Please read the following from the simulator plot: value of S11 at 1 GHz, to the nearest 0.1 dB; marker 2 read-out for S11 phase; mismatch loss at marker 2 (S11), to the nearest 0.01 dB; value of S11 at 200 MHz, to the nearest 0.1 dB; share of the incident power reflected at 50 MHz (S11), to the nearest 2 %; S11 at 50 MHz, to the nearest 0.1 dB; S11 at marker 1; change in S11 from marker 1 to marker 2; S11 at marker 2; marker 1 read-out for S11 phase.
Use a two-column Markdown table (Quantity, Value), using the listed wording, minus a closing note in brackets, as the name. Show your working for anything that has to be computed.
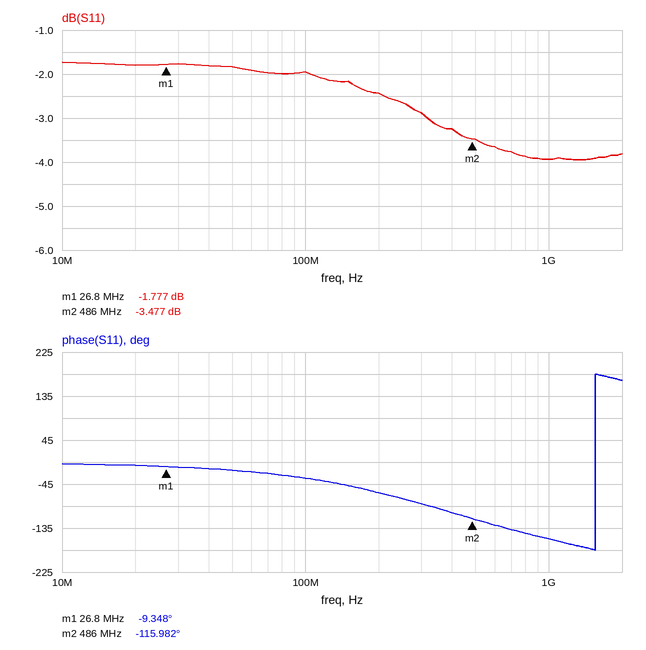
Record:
| Quantity | Value |
|---|---|
| value of S11 at 1 GHz, to the nearest 0.1 dB | -3.9 dB |
| marker 2 read-out for S11 phase | -115.982° |
| mismatch loss at marker 2 (S11), to the nearest 0.01 dB | −10 log10(1 − 10^(-3.477/10)) ≈ 2.59 dB |
| value of S11 at 200 MHz, to the nearest 0.1 dB | -2.4 dB |
| share of the incident power reflected at 50 MHz (S11), to the nearest 2 % | 10^(-1.8/10) ≈ 66 % |
| S11 at 50 MHz, to the nearest 0.1 dB | -1.8 dB |
| S11 at marker 1 | -1.777 dB |
| change in S11 from marker 1 to marker 2 | -3.477 − (-1.777) = -1.700 dB |
| S11 at marker 2 | -3.477 dB |
| marker 1 read-out for S11 phase | -9.348° |
